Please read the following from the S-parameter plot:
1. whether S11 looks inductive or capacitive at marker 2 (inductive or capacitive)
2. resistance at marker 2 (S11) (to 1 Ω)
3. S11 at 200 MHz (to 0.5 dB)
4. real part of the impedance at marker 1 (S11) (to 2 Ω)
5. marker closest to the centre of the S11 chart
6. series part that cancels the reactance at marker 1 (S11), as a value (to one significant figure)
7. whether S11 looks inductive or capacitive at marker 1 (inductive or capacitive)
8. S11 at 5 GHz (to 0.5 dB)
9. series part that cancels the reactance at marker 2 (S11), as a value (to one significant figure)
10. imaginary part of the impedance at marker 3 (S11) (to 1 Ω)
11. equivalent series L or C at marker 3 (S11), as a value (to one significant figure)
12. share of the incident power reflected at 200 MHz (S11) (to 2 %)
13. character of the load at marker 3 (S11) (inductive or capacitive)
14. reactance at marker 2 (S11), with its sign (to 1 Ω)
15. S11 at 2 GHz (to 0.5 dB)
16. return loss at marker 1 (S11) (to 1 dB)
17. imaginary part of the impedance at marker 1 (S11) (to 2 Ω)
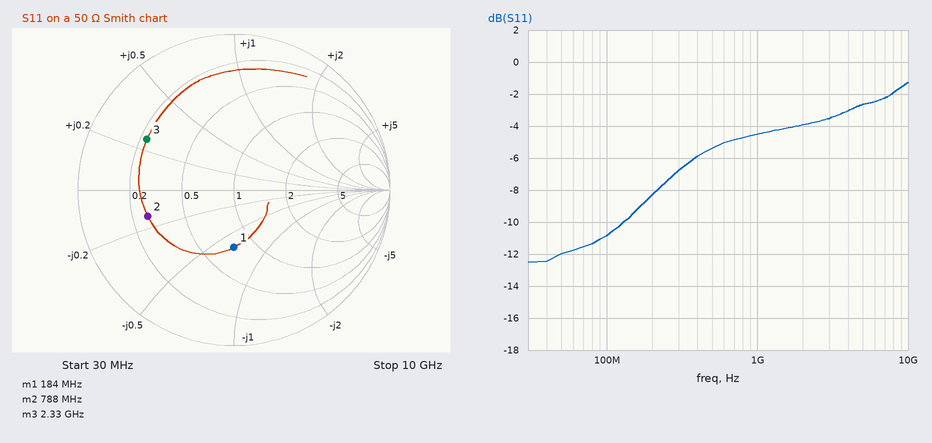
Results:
capacitive
14 Ω
-8.5 dB
38 Ω
marker 1
30 nH
capacitive
-2.5 dB
1 nH
+13 Ω
900 pH
14 %
inductive
-7 Ω
-4.0 dB
9 dB
-32 Ω
